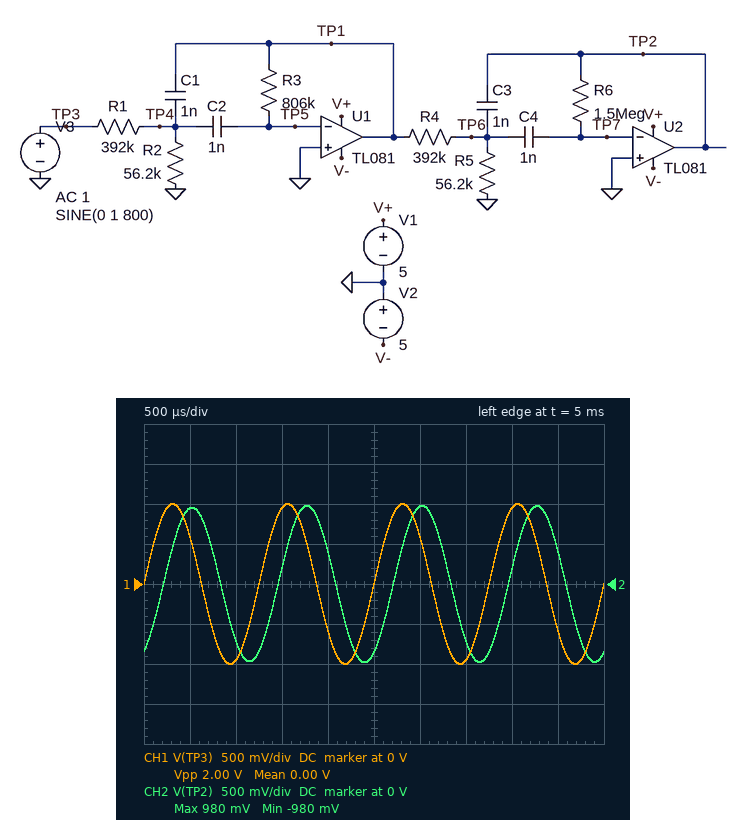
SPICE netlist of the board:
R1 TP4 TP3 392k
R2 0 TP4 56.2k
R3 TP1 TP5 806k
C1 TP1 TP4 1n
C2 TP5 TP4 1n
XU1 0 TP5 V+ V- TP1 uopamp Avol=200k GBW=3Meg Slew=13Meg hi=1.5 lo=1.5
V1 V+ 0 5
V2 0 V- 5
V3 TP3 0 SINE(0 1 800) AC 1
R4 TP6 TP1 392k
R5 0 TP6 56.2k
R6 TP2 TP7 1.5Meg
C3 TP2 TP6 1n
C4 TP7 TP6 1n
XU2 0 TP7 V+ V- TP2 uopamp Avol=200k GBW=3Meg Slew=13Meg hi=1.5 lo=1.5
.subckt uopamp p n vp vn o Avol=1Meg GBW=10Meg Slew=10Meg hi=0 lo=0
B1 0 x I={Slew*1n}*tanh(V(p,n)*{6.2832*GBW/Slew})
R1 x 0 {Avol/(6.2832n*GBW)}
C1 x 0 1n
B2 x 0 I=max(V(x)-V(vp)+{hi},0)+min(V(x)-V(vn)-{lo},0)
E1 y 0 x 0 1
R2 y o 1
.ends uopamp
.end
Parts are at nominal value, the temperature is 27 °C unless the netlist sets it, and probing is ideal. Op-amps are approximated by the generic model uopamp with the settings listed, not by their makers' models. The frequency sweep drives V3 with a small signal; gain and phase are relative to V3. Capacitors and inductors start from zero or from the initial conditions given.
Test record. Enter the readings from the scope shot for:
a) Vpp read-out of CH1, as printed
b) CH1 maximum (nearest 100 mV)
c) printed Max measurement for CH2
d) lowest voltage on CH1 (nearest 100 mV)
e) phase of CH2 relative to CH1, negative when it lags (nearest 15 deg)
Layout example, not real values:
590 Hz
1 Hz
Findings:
2.00 V
1.0 V
980 mV
-1.0 V
-60 deg
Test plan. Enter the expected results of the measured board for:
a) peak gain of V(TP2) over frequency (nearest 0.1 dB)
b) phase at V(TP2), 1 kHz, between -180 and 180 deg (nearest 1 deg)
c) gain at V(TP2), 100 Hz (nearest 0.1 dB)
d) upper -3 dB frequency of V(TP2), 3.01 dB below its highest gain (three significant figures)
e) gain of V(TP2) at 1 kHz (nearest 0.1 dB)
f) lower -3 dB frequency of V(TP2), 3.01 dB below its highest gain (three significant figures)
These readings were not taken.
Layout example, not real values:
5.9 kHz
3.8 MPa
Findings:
2.3 dB
-115 deg
-42.1 dB
816 Hz
-7.0 dB
538 Hz
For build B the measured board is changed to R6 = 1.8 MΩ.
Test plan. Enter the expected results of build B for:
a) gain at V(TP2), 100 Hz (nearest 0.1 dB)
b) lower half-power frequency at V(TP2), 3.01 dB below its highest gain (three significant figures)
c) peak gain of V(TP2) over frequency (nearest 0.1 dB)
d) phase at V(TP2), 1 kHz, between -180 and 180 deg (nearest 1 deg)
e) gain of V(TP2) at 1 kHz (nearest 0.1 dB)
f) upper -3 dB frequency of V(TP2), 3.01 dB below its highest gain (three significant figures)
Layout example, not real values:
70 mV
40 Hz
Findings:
-40.5 dB
490 Hz
2.2 dB
-119 deg
-7.6 dB
787 Hz
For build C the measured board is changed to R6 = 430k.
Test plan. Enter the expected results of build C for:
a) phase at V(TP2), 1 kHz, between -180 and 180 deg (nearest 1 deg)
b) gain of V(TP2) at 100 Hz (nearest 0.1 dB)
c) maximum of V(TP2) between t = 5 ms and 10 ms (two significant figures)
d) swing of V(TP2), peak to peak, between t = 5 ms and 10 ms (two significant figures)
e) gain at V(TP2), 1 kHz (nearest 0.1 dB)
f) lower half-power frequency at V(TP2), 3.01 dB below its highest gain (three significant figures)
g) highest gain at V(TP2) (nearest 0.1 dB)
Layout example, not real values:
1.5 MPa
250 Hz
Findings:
-28 deg
-53.2 dB
410 mV
820 mV
-7.9 dB
713 Hz
-7.1 dB
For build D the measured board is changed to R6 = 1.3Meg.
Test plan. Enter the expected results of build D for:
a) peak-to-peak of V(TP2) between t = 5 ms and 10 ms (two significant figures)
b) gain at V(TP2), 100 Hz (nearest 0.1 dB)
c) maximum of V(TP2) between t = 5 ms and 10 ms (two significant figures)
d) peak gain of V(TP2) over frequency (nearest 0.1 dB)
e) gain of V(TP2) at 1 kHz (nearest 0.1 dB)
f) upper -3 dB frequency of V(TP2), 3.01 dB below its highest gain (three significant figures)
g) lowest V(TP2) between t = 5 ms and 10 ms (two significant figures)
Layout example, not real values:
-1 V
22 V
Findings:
2.1 V
-43.4 dB
1.1 V
2.4 dB
-6.5 dB
837 Hz
-1.1 V
